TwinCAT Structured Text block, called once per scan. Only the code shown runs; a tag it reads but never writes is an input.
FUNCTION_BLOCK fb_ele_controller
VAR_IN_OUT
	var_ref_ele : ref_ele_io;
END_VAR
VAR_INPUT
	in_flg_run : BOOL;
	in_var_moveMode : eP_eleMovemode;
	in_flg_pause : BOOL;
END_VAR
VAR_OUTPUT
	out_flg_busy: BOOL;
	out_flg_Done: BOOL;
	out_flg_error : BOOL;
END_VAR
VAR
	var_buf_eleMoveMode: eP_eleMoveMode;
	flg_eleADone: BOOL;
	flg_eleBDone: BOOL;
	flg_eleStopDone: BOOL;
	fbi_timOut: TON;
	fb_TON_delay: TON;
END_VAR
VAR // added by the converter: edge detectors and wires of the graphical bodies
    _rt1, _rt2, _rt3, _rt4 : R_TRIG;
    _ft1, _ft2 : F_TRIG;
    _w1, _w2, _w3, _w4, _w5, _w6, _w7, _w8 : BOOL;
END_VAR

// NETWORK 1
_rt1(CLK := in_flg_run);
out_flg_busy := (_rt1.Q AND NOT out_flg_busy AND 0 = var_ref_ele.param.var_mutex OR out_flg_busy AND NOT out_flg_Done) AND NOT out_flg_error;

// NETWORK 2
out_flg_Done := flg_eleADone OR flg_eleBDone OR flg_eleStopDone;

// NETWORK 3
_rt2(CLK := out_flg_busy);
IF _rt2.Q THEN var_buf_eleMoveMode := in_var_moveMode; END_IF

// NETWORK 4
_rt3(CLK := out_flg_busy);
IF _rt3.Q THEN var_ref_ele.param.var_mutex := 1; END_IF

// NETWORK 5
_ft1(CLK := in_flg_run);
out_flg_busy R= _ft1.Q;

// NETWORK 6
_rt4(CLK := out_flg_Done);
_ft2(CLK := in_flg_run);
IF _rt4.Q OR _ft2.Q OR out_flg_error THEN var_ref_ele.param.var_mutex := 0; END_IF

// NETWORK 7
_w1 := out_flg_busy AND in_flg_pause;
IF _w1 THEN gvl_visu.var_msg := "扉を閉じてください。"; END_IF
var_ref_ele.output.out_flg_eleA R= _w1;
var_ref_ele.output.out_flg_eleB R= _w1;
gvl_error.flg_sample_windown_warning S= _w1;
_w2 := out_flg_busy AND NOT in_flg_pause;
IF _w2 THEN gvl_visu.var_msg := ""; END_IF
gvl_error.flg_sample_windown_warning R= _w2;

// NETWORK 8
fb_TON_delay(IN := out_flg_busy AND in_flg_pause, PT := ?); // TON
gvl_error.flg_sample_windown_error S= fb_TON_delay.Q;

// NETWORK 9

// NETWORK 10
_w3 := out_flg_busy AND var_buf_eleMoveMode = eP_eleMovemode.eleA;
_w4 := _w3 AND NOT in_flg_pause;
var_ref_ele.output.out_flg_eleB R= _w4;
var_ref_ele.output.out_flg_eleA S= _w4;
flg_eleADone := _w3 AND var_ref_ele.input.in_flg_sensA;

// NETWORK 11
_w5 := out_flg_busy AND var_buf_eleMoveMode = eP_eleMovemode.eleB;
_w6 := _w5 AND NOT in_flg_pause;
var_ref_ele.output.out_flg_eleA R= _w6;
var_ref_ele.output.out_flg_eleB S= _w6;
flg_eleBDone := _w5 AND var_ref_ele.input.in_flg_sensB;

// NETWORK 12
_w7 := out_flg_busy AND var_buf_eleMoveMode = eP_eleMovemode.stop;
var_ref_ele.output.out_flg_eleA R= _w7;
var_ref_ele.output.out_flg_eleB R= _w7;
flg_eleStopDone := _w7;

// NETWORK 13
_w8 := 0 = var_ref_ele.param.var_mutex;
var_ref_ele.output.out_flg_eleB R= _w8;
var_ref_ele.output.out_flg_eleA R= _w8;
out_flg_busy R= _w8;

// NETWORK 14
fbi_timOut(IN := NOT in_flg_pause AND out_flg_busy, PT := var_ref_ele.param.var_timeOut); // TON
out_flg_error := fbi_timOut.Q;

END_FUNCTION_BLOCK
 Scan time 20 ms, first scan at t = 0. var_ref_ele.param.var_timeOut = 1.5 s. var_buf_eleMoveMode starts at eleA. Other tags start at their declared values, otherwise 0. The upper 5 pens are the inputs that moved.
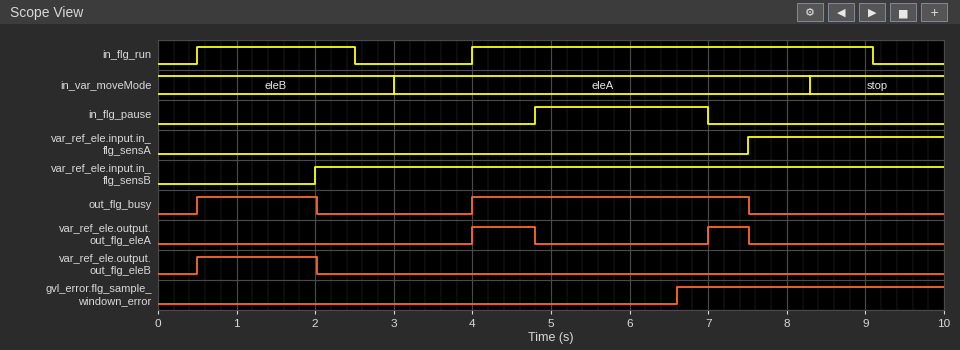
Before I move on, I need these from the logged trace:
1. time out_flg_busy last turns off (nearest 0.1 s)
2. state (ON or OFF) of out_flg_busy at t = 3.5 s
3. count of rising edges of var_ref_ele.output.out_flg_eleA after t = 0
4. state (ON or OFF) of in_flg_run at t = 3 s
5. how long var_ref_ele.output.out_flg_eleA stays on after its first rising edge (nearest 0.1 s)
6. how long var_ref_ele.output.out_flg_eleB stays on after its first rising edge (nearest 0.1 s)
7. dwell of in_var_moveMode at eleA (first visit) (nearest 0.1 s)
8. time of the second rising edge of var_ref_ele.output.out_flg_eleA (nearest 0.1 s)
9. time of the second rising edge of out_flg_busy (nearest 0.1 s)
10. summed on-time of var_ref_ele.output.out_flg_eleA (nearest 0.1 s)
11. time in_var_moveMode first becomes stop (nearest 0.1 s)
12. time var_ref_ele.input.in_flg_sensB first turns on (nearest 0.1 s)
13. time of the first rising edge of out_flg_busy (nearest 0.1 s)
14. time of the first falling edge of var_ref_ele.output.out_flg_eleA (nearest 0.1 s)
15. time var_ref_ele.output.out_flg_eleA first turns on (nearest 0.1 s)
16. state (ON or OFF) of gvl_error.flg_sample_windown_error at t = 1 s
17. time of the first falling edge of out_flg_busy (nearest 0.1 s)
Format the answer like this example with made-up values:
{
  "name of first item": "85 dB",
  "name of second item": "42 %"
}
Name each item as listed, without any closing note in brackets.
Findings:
{
  "time out_flg_busy last turns off": "7.5 s",
  "state (ON or OFF) of out_flg_busy at t = 3.5 s": "OFF",
  "count of rising edges of var_ref_ele.output.out_flg_eleA after t = 0": "2",
  "state (ON or OFF) of in_flg_run at t = 3 s": "OFF",
  "how long var_ref_ele.output.out_flg_eleA stays on after its first rising edge": "0.8 s",
  "how long var_ref_ele.output.out_flg_eleB stays on after its first rising edge": "1.5 s",
  "dwell of in_var_moveMode at eleA (first visit)": "5.3 s",
  "time of the second rising edge of var_ref_ele.output.out_flg_eleA": "7.0 s",
  "time of the second rising edge of out_flg_busy": "4.0 s",
  "summed on-time of var_ref_ele.output.out_flg_eleA": "1.3 s",
  "time in_var_moveMode first becomes stop": "8.3 s",
  "time var_ref_ele.input.in_flg_sensB first turns on": "2.0 s",
  "time of the first rising edge of out_flg_busy": "0.5 s",
  "time of the first falling edge of var_ref_ele.output.out_flg_eleA": "4.8 s",
  "time var_ref_ele.output.out_flg_eleA first turns on": "4.0 s",
  "state (ON or OFF) of gvl_error.flg_sample_windown_error at t = 1 s": "OFF",
  "time of the first falling edge of out_flg_busy": "2.0 s"
}
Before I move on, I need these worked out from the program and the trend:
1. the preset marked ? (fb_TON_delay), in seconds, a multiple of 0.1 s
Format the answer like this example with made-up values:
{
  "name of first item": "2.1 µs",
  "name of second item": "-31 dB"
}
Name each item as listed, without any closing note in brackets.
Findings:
{
  "the preset marked ? (fb_TON_delay), in seconds, a multiple of 0.1 s": "1.8 s"
}
